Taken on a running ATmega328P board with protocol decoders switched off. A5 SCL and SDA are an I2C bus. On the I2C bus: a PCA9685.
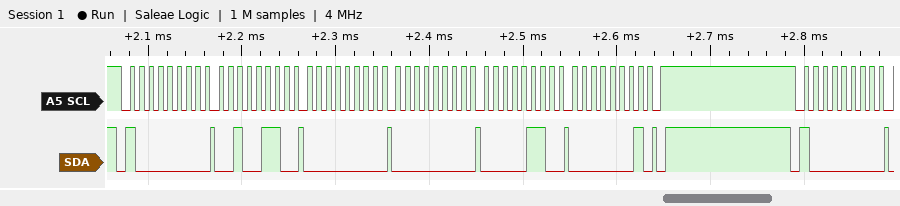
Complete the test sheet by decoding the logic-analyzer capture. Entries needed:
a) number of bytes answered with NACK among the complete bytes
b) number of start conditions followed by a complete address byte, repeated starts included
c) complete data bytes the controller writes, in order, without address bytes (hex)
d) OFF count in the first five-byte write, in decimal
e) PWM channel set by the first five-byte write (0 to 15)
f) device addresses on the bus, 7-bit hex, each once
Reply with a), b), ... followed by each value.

a) 0
b) 2
c) 26 00 00 06 01
d) 262
e) 8
f) 0x40
